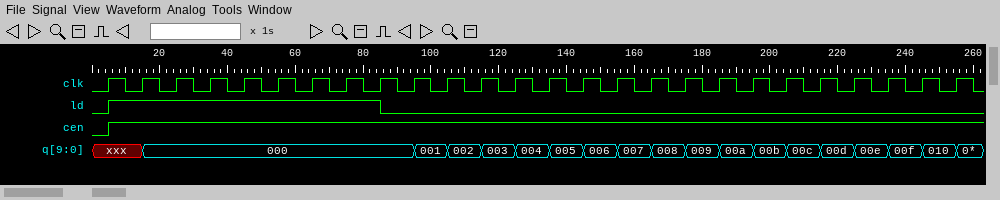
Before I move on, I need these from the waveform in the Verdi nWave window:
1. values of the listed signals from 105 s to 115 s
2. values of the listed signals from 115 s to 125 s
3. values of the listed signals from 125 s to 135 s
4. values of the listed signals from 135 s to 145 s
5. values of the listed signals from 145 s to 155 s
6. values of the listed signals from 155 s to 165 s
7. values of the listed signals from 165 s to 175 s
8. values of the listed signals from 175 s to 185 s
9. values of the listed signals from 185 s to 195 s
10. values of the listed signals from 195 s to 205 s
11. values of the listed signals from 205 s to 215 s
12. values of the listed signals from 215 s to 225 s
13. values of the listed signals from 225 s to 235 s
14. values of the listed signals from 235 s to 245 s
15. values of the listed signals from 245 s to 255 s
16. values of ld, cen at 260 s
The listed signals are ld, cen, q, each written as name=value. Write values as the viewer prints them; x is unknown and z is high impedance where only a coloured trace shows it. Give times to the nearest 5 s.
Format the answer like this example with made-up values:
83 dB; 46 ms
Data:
ld=0, cen=1, q=002; ld=0, cen=1, q=003; ld=0, cen=1, q=004; ld=0, cen=1, q=005; ld=0, cen=1, q=006; ld=0, cen=1, q=007; ld=0, cen=1, q=008; ld=0, cen=1, q=009; ld=0, cen=1, q=00a; ld=0, cen=1, q=00b; ld=0, cen=1, q=00c; ld=0, cen=1, q=00d; ld=0, cen=1, q=00e; ld=0, cen=1, q=00f; ld=0, cen=1, q=010; ld=0, cen=1
